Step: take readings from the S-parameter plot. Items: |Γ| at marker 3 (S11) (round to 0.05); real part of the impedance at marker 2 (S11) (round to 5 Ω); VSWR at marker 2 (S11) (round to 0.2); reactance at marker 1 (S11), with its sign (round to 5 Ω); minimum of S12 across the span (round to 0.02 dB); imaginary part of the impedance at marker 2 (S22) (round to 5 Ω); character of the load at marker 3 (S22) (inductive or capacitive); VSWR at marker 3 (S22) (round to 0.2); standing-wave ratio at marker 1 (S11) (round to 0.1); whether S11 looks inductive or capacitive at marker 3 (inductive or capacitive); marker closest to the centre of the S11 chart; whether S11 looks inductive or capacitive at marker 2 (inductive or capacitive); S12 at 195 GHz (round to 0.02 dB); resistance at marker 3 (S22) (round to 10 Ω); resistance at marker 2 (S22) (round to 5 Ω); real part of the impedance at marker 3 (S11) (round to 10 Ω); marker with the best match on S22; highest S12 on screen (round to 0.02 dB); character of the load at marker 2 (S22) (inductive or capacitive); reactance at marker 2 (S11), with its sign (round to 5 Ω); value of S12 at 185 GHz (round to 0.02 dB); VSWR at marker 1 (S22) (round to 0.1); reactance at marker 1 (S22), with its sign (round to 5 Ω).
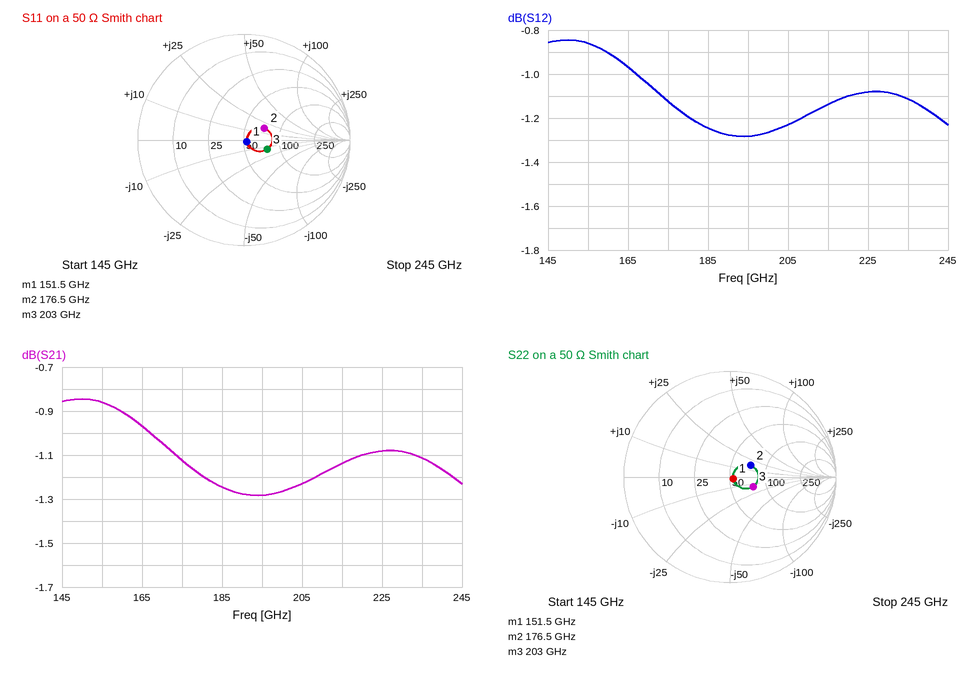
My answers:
0.25
70 Ω
1.6
0 Ω
-1.28 dB
+15 Ω
capacitive
1.6
1.1
capacitive
marker 1
inductive
-1.28 dB
80 Ω
70 Ω
80 Ω
marker 1
-0.84 dB
inductive
+15 Ω
-1.24 dB
1.1
0 Ω
